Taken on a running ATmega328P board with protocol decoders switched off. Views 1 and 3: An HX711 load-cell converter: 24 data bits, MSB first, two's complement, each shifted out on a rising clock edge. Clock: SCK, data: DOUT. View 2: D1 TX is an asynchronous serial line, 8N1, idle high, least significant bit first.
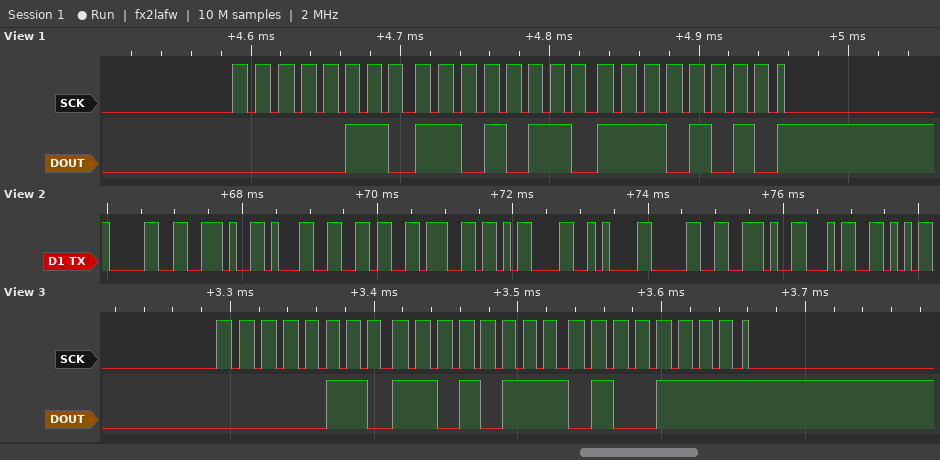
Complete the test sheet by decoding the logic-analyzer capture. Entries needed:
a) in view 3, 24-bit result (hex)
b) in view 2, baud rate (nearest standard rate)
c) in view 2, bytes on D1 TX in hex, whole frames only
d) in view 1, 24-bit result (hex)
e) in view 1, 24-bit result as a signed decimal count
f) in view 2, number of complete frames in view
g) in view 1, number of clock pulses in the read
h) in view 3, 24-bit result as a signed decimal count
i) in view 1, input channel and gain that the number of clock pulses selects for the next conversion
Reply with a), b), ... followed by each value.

a) 0x06D74F
b) 9600 baud
c) 30 2E 31 36 67 0D 0A 30 2E 34
d) 0x06D6EA
e) 448234
f) 10
g) 25
h) 448335
i) channel A, gain 128
